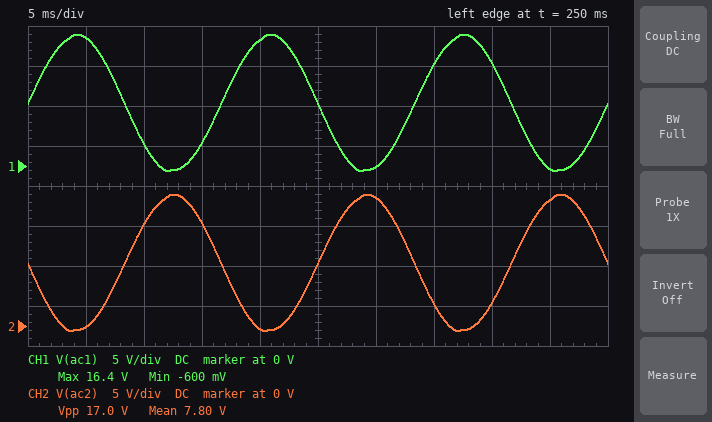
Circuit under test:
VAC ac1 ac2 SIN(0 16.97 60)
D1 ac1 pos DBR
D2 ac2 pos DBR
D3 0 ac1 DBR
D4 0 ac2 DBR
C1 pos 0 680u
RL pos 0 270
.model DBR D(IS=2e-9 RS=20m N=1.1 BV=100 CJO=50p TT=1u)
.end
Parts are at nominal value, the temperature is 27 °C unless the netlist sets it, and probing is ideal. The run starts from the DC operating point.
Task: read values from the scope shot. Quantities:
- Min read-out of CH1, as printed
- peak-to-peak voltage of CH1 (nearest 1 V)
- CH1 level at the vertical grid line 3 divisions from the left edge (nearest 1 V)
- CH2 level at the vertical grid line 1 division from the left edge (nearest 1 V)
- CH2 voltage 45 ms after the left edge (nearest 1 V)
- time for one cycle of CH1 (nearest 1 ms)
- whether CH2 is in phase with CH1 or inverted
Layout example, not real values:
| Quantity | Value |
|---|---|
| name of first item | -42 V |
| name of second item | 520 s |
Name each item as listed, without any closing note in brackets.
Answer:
| Quantity | Value |
|---|---|
| Min read-out of CH1, as printed | -600 mV |
| peak-to-peak voltage of CH1 | 17 V |
| CH1 level at the vertical grid line 3 divisions from the left edge | 3 V |
| CH2 level at the vertical grid line 1 division from the left edge | 0 V |
| CH2 voltage 45 ms after the left edge | 16 V |
| time for one cycle of CH1 | 17 ms |
| whether CH2 is in phase with CH1 or inverted | inverted |
